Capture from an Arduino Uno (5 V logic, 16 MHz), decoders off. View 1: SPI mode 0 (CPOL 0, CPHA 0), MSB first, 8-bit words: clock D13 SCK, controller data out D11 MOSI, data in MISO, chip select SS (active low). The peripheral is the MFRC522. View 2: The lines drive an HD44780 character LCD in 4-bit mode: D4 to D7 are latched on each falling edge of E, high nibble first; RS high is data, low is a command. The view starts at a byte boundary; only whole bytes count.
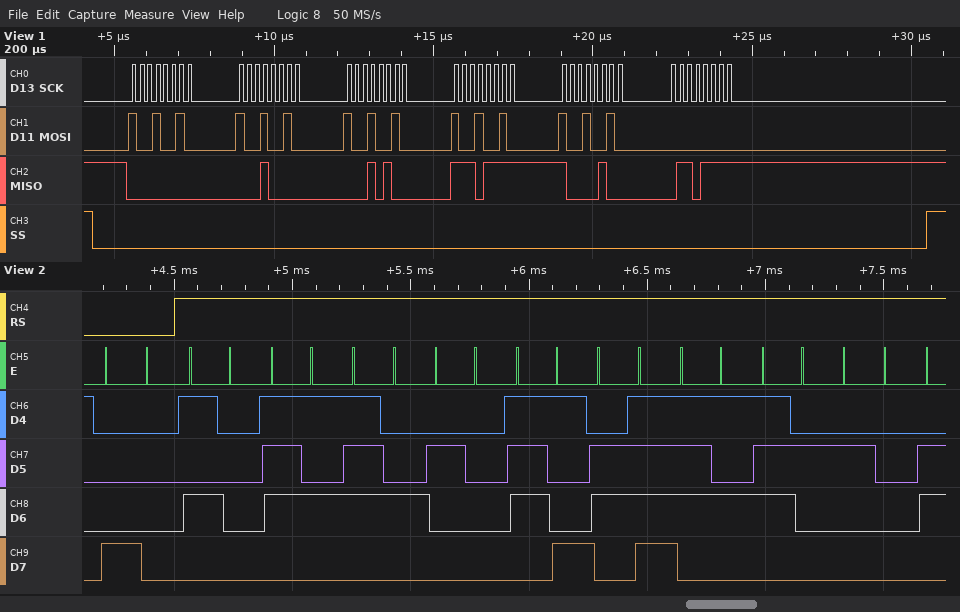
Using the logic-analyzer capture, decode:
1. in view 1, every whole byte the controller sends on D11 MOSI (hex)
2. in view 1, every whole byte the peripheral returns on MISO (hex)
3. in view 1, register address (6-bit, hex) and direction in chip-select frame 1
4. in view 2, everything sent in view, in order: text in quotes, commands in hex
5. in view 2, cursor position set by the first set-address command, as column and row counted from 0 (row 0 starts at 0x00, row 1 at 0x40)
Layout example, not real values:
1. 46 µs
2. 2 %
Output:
1. 92 92 92 92 92 00
2. 00 10 14 EF 84 6F
3. 0x09 read
4. 0x80 "Put your "
5. column 0, row 0
